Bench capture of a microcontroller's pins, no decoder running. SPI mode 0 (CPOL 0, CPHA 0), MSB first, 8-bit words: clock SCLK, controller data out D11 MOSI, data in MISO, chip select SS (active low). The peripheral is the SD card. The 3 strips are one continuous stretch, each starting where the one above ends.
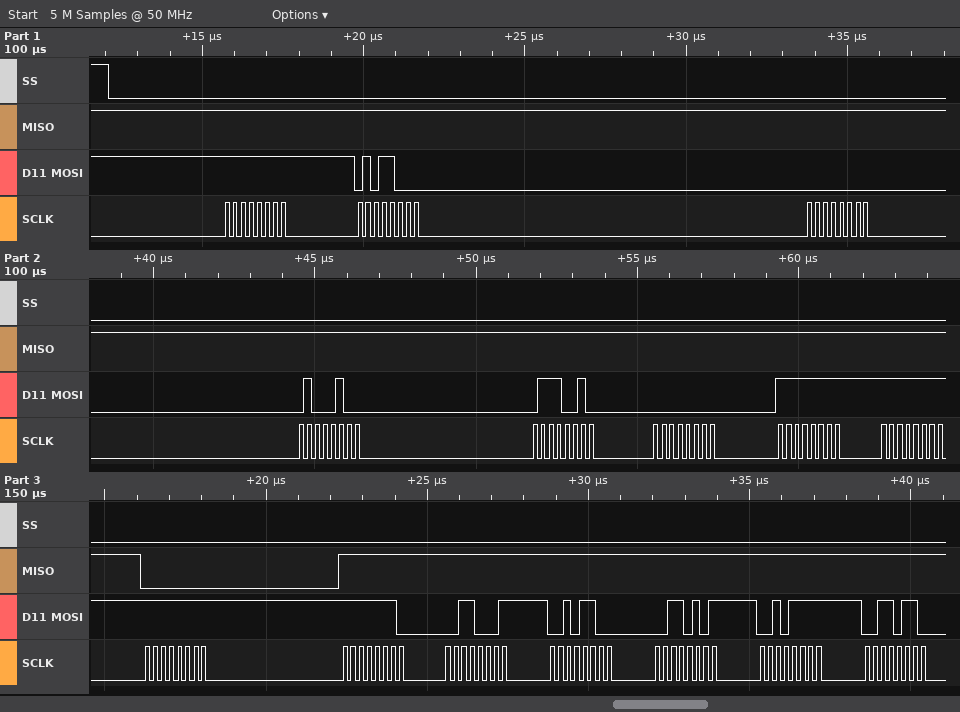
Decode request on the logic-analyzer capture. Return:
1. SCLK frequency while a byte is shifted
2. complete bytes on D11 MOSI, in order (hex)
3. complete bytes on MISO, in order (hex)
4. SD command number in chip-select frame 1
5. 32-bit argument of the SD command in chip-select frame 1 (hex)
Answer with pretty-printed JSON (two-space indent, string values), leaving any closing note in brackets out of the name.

{
  "SCLK frequency while a byte is shifted": "4 MHz",
  "complete bytes on D11 MOSI, in order": "0xFF 0x58 0x00 0x44 0x72 0x00 0xFF 0xFF 0xFF 0xFE 0x31 0x2C 0x35 0x2F 0x36",
  "complete bytes on MISO, in order": "0xFF 0xFF 0xFF 0xFF 0xFF 0xFF 0xFF 0xFF 0x00 0xFF 0xFF 0xFF 0xFF 0xFF 0xFF",
  "SD command number in chip-select frame 1": "CMD24",
  "32-bit argument of the SD command in chip-select frame 1": "0x00447200"
}
